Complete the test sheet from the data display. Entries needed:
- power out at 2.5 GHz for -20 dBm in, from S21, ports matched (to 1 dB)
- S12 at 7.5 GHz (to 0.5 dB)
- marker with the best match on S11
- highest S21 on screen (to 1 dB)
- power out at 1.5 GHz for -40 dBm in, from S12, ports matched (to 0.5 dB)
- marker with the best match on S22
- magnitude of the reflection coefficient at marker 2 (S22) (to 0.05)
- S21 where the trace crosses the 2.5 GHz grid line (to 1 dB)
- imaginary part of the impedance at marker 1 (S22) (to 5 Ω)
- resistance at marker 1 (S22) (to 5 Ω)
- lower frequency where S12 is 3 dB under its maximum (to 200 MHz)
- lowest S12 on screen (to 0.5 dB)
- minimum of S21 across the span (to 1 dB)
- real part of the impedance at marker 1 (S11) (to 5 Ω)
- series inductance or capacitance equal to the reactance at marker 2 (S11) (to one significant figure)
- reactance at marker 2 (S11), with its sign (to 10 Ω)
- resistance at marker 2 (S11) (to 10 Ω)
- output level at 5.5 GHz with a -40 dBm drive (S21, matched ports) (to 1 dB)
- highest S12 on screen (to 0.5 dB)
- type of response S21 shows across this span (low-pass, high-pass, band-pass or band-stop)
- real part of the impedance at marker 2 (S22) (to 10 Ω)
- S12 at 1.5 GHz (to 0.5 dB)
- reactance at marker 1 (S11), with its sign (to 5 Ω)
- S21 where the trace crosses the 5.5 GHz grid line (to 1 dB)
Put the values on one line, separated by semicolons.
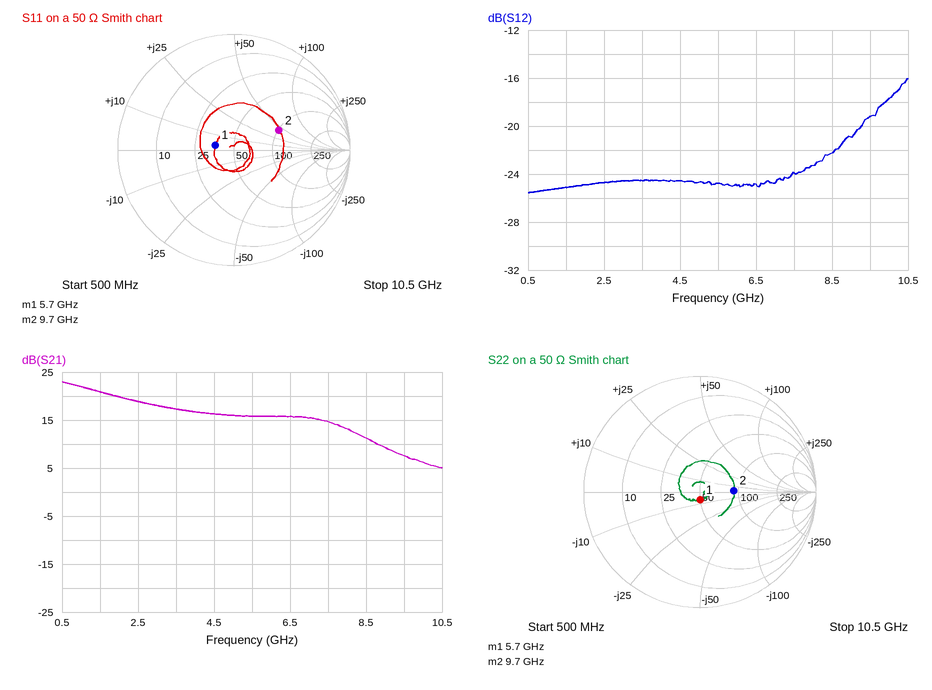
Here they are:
-1 dBm; -24.0 dB; marker 1; 23 dB; -65.0 dBm; marker 1; 0.30; 19 dB; -5 Ω; 50 Ω; 9.6 GHz; -25.5 dB; 5 dB; 35 Ω; 700 pH; +40 Ω; 100 Ω; -24 dBm; -16.0 dB; low-pass; 90 Ω; -25.0 dB; +5 Ω; 16 dB
